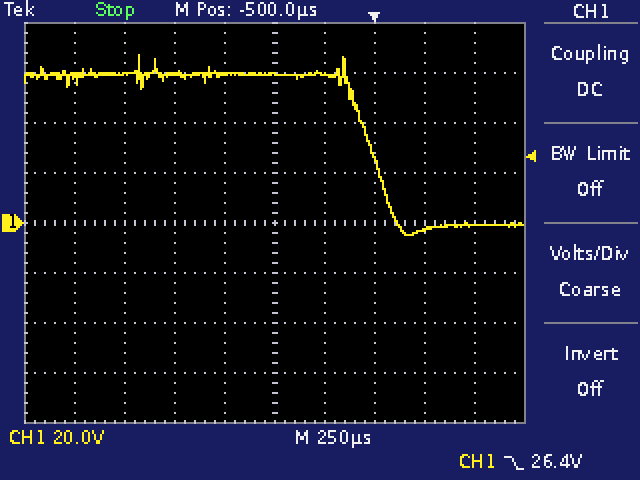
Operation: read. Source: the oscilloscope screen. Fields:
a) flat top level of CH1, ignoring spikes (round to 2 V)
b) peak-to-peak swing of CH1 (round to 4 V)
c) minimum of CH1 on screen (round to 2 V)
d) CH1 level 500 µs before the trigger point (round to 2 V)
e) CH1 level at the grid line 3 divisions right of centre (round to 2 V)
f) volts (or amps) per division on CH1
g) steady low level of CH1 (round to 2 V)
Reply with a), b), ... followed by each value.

a) 60 V
b) 72 V
c) -4 V
d) 60 V
e) -2 V
f) 20 V
g) 0 V
